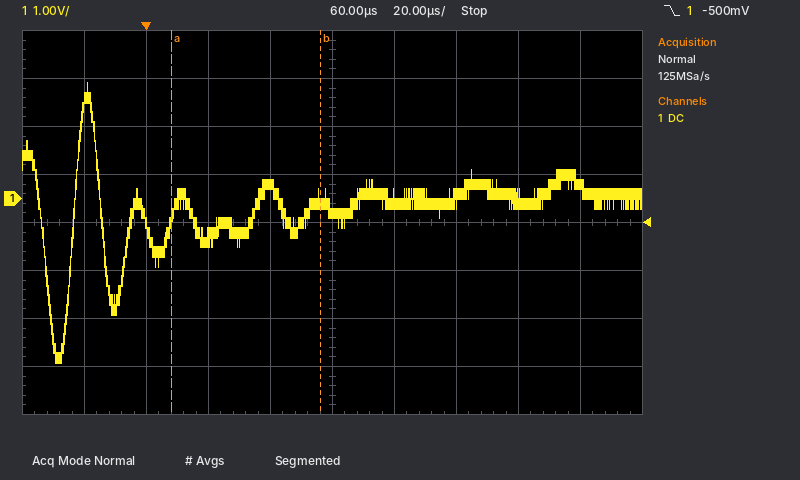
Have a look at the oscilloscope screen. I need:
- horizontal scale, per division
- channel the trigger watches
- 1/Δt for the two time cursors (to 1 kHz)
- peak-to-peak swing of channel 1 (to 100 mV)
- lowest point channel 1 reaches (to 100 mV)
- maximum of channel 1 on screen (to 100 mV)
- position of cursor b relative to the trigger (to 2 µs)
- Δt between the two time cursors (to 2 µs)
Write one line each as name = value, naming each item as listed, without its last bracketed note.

horizontal scale, per division = 20 µs
channel the trigger watches = channel 1
1/Δt for the two time cursors = 21 kHz
peak-to-peak swing of channel 1 = 5.8 V
lowest point channel 1 reaches = -3.4 V
maximum of channel 1 on screen = 2.4 V
position of cursor b relative to the trigger = +56 µs
Δt between the two time cursors = 48 µs
